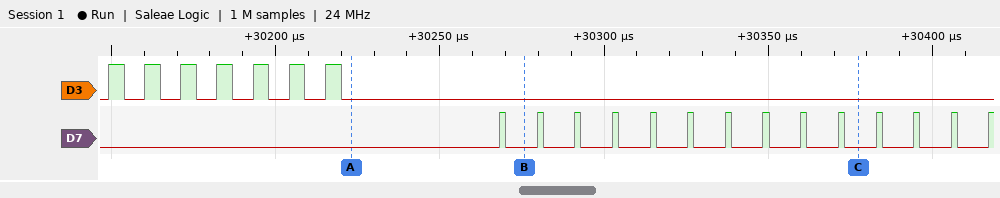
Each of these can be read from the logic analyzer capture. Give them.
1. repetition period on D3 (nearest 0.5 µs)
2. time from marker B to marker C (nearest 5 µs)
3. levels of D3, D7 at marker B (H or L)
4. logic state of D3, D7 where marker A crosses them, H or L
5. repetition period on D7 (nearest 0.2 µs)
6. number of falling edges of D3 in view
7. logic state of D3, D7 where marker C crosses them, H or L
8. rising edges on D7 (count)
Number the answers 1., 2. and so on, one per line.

1. 11 µs
2. 100 µs
3. D3=L, D7=L
4. D3=L, D7=L
5. 11.4 µs
6. 7
7. D3=L, D7=L
8. 14
